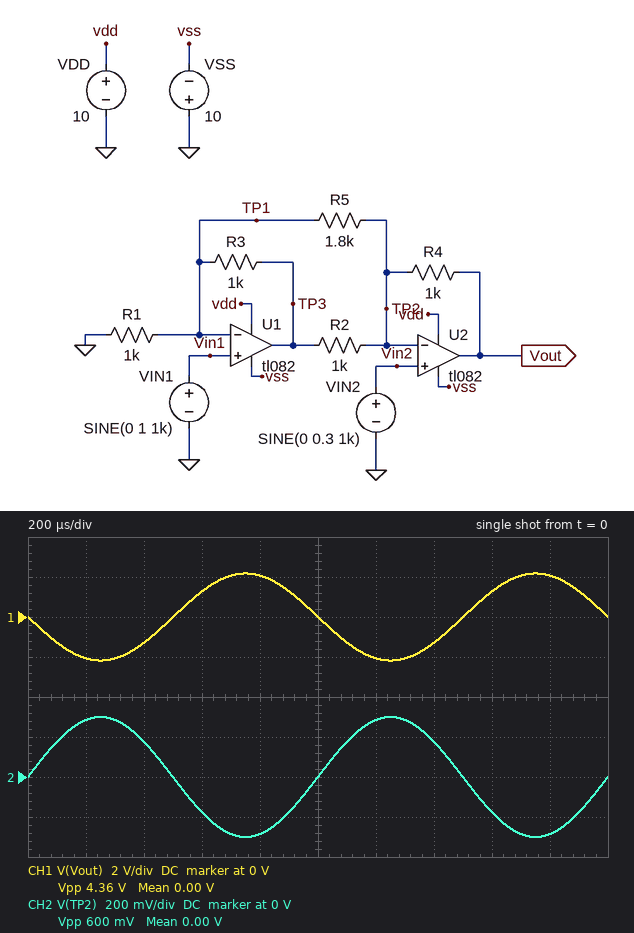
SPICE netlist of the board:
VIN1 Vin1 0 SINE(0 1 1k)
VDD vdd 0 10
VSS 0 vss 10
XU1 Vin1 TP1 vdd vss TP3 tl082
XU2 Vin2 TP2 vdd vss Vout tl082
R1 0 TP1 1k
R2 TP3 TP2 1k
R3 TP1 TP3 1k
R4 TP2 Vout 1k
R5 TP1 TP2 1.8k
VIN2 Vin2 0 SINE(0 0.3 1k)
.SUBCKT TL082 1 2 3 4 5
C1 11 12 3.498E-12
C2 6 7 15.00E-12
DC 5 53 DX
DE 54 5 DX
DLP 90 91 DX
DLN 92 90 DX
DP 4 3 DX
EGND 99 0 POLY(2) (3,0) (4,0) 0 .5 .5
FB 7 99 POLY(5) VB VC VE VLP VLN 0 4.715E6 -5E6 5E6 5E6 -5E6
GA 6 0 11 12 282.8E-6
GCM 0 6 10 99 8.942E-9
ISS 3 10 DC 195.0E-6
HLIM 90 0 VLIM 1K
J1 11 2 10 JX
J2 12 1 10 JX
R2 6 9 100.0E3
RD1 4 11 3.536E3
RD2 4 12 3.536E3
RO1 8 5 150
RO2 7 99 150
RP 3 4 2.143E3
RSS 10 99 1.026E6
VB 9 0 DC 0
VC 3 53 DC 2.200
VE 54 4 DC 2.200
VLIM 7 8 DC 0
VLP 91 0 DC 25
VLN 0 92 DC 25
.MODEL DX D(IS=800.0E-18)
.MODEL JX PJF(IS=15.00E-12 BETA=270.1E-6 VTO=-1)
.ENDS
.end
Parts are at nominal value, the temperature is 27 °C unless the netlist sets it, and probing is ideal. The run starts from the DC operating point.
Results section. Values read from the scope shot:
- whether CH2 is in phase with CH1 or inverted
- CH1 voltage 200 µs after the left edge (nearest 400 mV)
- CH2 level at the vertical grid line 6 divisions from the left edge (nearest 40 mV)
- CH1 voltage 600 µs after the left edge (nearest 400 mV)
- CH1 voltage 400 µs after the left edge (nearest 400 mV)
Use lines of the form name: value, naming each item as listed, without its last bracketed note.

whether CH2 is in phase with CH1 or inverted: inverted
CH1 voltage 200 µs after the left edge: -2.0 V
CH2 level at the vertical grid line 6 divisions from the left edge: 280 mV
CH1 voltage 600 µs after the left edge: 1.2 V
CH1 voltage 400 µs after the left edge: -1.2 V
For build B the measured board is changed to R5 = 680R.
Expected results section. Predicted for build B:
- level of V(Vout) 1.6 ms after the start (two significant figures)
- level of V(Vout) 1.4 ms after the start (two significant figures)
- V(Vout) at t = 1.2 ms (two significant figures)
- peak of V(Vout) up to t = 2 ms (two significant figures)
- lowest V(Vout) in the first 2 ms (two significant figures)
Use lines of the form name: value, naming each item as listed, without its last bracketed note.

level of V(Vout) 1.6 ms after the start: 2.0 V
level of V(Vout) 1.4 ms after the start: -2.0 V
V(Vout) at t = 1.2 ms: -3.3 V
peak of V(Vout) up to t = 2 ms: 3.5 V
lowest V(Vout) in the first 2 ms: -3.5 V
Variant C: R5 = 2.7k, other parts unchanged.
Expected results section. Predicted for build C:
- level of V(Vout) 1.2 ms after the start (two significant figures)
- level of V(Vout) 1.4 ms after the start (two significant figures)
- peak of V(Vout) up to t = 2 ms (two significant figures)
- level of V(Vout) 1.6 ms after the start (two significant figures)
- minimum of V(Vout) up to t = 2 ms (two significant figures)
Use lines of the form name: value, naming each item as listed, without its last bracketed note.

level of V(Vout) 1.2 ms after the start: -1.8 V
level of V(Vout) 1.4 ms after the start: -1.1 V
peak of V(Vout) up to t = 2 ms: 1.9 V
level of V(Vout) 1.6 ms after the start: 1.1 V
minimum of V(Vout) up to t = 2 ms: -1.9 V
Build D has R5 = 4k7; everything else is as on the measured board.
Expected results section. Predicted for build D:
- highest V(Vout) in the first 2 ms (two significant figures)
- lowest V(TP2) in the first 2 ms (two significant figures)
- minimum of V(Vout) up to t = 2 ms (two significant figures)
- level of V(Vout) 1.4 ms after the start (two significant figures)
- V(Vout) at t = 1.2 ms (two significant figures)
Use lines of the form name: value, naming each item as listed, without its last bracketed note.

highest V(Vout) in the first 2 ms: 1.7 V
lowest V(TP2) in the first 2 ms: -300 mV
minimum of V(Vout) up to t = 2 ms: -1.7 V
level of V(Vout) 1.4 ms after the start: -1.0 V
V(Vout) at t = 1.2 ms: -1.6 V
